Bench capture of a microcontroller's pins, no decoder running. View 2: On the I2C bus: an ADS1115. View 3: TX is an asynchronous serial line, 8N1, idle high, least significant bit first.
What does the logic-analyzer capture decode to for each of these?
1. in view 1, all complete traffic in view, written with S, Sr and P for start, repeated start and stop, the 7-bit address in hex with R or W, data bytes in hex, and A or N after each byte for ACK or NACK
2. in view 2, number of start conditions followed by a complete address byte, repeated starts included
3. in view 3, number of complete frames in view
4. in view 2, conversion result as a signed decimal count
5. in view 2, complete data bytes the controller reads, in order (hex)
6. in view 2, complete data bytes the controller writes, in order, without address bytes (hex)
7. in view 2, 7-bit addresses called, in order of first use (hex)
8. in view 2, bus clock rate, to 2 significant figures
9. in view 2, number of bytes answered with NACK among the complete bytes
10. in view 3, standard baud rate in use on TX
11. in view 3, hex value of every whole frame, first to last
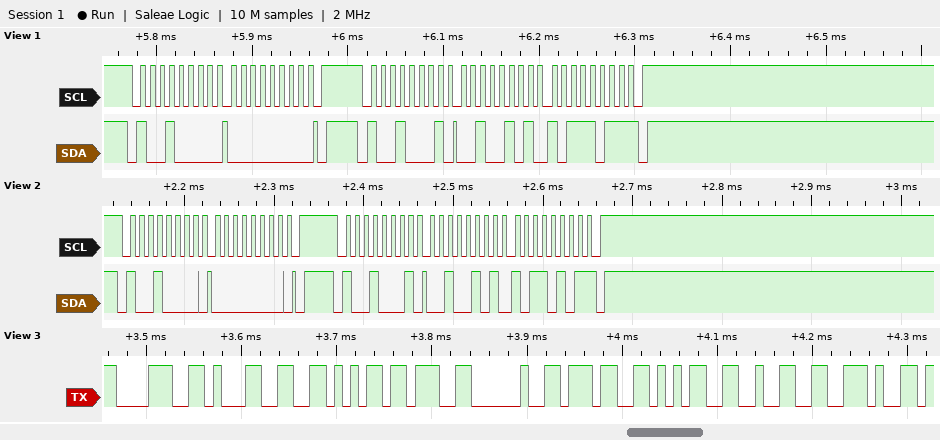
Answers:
S 48W A 00 A P S 48R A 25 A BB N P
2
9
9653
25 B5
00
0x48
100 kHz
1
115200 baud
38 31 56 3B 20 37 35 32 2E
